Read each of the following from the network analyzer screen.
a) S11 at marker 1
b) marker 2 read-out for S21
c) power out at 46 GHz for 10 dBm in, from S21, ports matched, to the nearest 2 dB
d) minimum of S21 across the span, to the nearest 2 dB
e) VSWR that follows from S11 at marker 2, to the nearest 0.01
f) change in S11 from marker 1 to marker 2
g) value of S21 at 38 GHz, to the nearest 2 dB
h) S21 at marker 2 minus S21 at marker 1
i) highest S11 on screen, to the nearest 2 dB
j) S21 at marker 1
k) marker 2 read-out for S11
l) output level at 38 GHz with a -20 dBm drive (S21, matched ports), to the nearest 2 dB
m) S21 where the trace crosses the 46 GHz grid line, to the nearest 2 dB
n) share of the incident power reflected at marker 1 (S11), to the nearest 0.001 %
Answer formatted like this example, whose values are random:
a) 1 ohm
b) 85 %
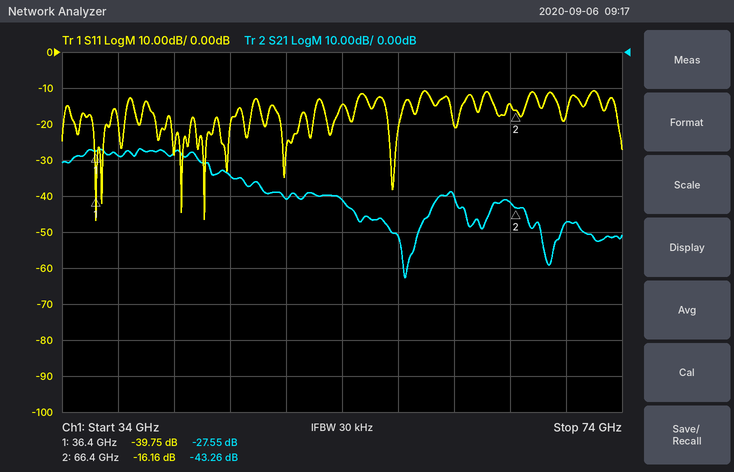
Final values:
a) -39.75 dB
b) -43.26 dB
c) -24 dBm
d) -62 dB
e) 1.37
f) 23.59 dB
g) -28 dB
h) -15.71 dB
i) -10 dB
j) -27.55 dB
k) -16.16 dB
l) -48 dBm
m) -34 dB
n) 0.011 %
